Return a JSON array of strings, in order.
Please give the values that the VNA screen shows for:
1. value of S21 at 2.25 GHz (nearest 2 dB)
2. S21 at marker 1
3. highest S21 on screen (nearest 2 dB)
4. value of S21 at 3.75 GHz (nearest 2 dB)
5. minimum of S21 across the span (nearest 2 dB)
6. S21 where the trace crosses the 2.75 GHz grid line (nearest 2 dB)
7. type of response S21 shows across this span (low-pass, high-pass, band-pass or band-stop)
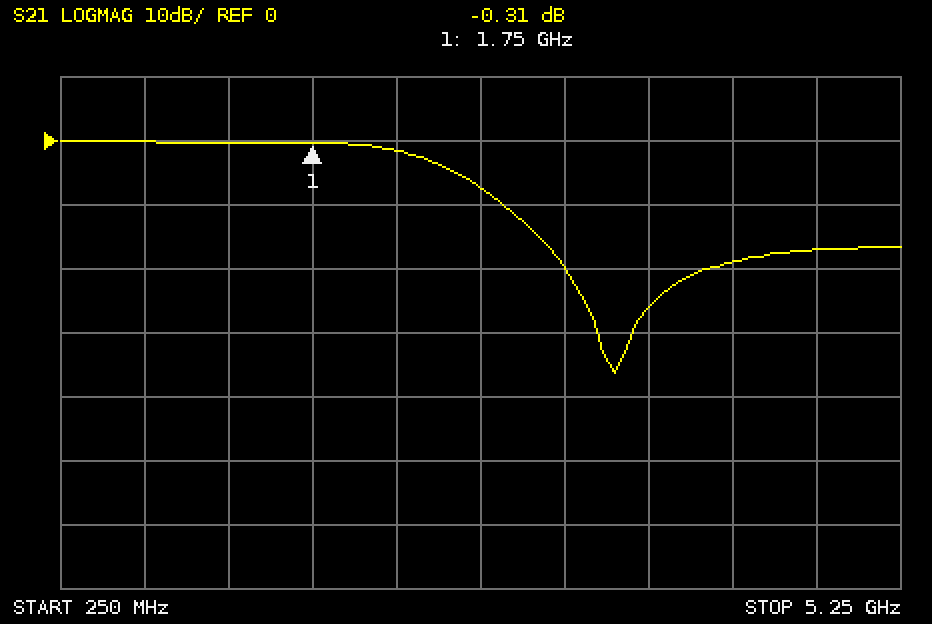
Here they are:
["-2 dB", "-0.31 dB", "0 dB", "-26 dB", "-36 dB", "-8 dB", "low-pass"]
